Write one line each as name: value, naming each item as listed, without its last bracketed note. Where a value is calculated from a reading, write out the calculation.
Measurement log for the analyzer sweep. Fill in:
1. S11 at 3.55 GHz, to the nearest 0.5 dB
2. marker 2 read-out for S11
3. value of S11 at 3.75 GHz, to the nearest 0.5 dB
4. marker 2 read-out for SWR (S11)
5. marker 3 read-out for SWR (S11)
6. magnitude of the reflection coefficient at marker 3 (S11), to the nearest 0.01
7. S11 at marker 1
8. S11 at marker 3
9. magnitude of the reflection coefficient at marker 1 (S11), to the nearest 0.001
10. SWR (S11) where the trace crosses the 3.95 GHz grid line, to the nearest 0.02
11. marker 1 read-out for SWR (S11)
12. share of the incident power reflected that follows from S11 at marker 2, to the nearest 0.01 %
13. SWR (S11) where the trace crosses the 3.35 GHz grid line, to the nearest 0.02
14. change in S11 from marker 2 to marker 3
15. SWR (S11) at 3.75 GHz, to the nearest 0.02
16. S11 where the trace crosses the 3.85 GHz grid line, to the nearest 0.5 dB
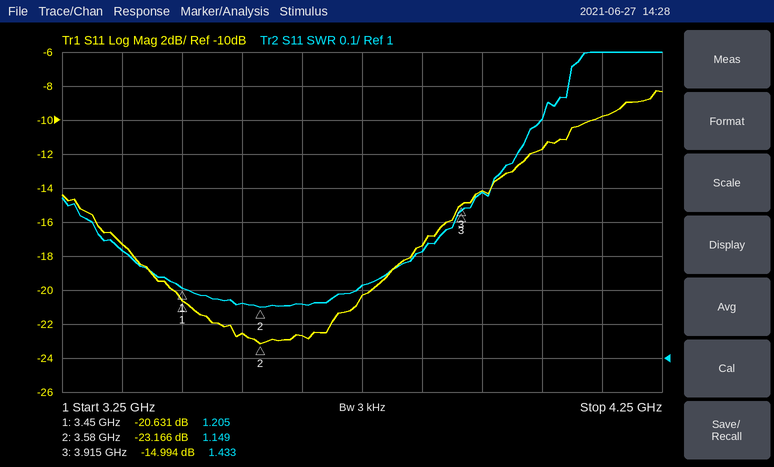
S11 at 3.55 GHz, to the nearest 0.5 dB: -22.5 dB
marker 2 read-out for S11: -23.166 dB
value of S11 at 3.75 GHz, to the nearest 0.5 dB: -20.5 dB
marker 2 read-out for SWR: 1.149
marker 3 read-out for SWR: 1.433
magnitude of the reflection coefficient at marker 3 (S11), to the nearest 0.01: 10^(-14.994/20) ≈ 0.18
S11 at marker 1: -20.631 dB
S11 at marker 3: -14.994 dB
magnitude of the reflection coefficient at marker 1 (S11), to the nearest 0.001: 10^(-20.631/20) ≈ 0.093
SWR (S11) where the trace crosses the 3.95 GHz grid line, to the nearest 0.02: 1.48
marker 1 read-out for SWR: 1.205
share of the incident power reflected that follows from S11 at marker 2, to the nearest 0.01 %: 10^(-23.166/10) ≈ 0.48 %
SWR (S11) where the trace crosses the 3.35 GHz grid line, to the nearest 0.02: 1.32
change in S11 from marker 2 to marker 3: -14.994 − (-23.166) = 8.172 dB
SWR (S11) at 3.75 GHz, to the nearest 0.02: 1.22
S11 where the trace crosses the 3.85 GHz grid line, to the nearest 0.5 dB: -17.5 dB
